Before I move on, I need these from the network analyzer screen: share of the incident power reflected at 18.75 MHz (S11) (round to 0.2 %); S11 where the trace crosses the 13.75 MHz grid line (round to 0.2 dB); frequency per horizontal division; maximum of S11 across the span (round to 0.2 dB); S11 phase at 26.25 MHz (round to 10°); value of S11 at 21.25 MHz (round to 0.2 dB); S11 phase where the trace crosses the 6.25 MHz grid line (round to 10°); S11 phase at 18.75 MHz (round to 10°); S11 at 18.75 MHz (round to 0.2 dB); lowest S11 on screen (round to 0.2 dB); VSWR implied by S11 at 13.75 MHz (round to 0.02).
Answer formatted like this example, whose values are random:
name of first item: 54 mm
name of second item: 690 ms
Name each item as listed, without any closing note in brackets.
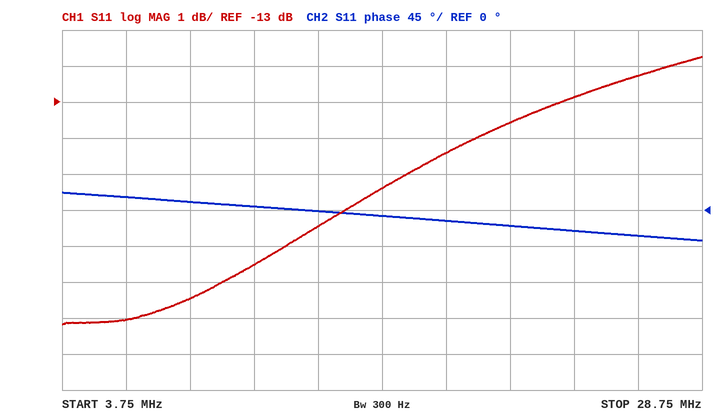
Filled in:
share of the incident power reflected at 18.75 MHz (S11): 3.6 %
S11 where the trace crosses the 13.75 MHz grid line: -16.4 dB
frequency per horizontal division: 2.5 MHz
maximum of S11 across the span: -11.8 dB
S11 phase at 26.25 MHz: -30°
value of S11 at 21.25 MHz: -13.6 dB
S11 phase where the trace crosses the 6.25 MHz grid line: 20°
S11 phase at 18.75 MHz: -10°
S11 at 18.75 MHz: -14.4 dB
lowest S11 on screen: -19.2 dB
VSWR implied by S11 at 13.75 MHz: 1.36
